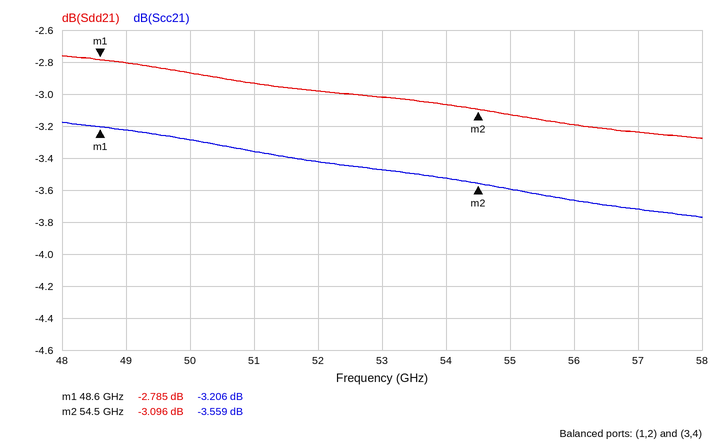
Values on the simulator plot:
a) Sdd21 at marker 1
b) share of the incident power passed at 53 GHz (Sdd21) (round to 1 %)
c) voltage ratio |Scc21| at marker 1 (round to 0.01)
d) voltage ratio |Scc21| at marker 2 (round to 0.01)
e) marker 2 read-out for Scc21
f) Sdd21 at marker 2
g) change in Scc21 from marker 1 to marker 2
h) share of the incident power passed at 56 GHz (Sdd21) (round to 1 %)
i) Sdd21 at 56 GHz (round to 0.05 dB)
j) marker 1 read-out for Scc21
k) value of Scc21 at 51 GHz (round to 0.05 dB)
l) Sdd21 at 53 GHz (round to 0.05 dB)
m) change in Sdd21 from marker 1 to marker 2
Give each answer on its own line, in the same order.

-2.785 dB
50 %
0.69
0.66
-3.559 dB
-3.096 dB
-0.353 dB
48 %
-3.20 dB
-3.206 dB
-3.35 dB
-3.00 dB
-0.311 dB
